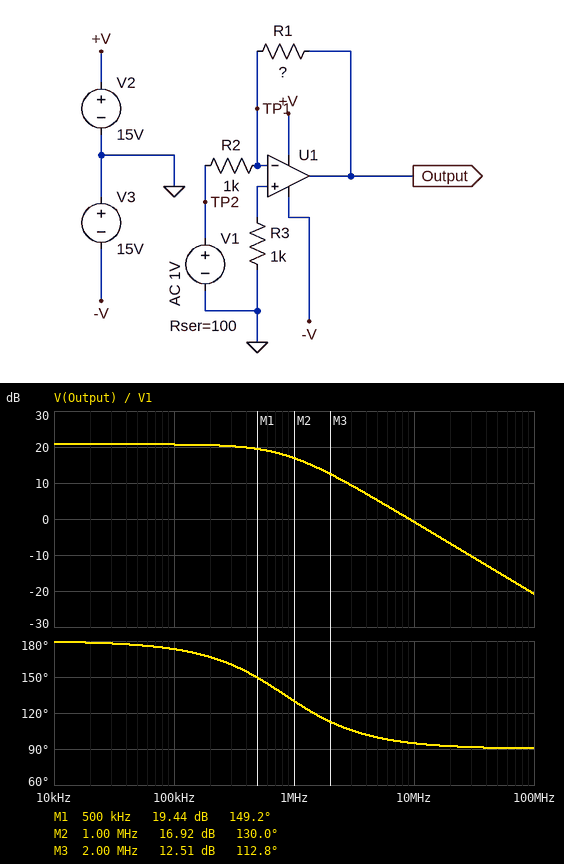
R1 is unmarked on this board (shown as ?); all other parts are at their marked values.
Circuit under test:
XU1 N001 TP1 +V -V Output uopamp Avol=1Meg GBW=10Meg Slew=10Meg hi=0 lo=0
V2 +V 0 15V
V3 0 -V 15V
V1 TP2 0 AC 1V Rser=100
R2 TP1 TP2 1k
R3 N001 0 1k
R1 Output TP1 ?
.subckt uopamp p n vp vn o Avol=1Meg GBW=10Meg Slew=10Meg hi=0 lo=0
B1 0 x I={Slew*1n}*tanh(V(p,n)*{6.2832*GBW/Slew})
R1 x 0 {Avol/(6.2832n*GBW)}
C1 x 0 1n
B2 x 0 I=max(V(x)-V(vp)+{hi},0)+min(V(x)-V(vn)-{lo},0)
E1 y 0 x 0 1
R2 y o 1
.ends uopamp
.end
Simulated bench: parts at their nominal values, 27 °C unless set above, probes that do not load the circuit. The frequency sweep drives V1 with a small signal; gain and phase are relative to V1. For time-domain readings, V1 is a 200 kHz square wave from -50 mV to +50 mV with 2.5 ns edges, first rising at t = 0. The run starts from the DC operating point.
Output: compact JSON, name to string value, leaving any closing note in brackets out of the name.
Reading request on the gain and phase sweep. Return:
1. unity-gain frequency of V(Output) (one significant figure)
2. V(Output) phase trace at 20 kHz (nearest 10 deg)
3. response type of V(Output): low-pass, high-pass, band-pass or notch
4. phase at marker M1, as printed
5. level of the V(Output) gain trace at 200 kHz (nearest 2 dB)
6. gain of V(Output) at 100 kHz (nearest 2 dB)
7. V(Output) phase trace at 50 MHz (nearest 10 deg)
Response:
{"unity-gain frequency of V(Output)": "9 MHz", "V(Output) phase trace at 20 kHz": "180 deg", "response type of V(Output): low-pass, high-pass, band-pass or notch": "low-pass", "phase at marker M1, as printed": "149.2 deg", "level of the V(Output) gain trace at 200 kHz": "20 dB", "gain of V(Output) at 100 kHz": "20 dB", "V(Output) phase trace at 50 MHz": "90 deg"}
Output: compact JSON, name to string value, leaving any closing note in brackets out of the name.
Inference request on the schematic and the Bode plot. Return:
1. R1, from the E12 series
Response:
{"R1, from the E12 series": "12 kΩ"}
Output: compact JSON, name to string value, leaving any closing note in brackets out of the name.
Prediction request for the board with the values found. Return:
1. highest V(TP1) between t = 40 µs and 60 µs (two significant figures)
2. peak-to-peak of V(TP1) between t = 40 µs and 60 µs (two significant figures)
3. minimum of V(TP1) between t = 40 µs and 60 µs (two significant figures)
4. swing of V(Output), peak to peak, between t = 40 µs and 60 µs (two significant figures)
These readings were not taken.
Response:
{"highest V(TP1) between t = 40 µs and 60 µs": "91 mV", "peak-to-peak of V(TP1) between t = 40 µs and 60 µs": "180 mV", "minimum of V(TP1) between t = 40 µs and 60 µs": "-91 mV", "swing of V(Output), peak to peak, between t = 40 µs and 60 µs": "1.1 V"}
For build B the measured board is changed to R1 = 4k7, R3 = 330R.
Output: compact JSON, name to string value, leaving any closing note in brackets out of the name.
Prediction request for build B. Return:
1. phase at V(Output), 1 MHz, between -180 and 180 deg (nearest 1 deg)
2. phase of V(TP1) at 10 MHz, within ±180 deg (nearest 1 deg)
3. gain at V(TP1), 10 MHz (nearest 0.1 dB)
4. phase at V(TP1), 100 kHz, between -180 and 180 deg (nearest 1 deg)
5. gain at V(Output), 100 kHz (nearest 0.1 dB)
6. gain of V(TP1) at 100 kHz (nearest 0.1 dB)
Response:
{"phase at V(Output), 1 MHz, between -180 and 180 deg": "152 deg", "phase of V(TP1) at 10 MHz, within ±180 deg": "11 deg", "gain at V(TP1), 10 MHz": "-2.0 dB", "phase at V(TP1), 100 kHz, between -180 and 180 deg": "87 deg", "gain at V(Output), 100 kHz": "12.6 dB", "gain of V(TP1) at 100 kHz": "-27.4 dB"}
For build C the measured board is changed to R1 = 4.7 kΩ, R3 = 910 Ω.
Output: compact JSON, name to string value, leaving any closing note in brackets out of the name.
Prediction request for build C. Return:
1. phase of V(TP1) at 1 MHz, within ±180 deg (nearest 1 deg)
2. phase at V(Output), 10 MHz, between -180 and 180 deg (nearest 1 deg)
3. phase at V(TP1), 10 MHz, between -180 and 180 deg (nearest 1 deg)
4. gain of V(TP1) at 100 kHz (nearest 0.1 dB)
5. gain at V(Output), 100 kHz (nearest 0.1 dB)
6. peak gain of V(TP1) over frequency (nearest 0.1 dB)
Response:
{"phase of V(TP1) at 1 MHz, within ±180 deg": "62 deg", "phase at V(Output), 10 MHz, between -180 and 180 deg": "101 deg", "phase at V(TP1), 10 MHz, between -180 and 180 deg": "11 deg", "gain of V(TP1) at 100 kHz": "-27.4 dB", "gain at V(Output), 100 kHz": "12.6 dB", "peak gain of V(TP1) over frequency": "-1.8 dB"}
